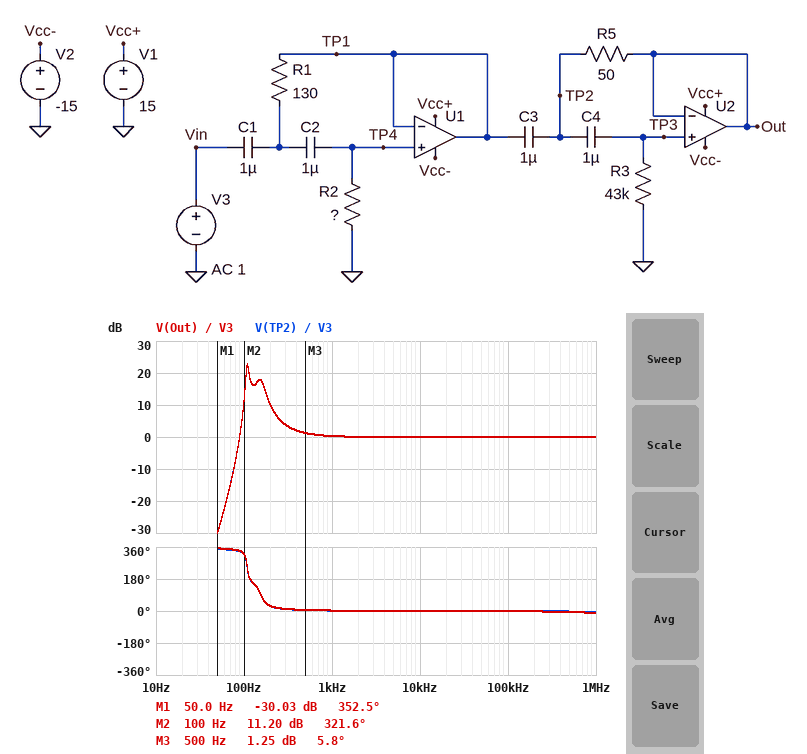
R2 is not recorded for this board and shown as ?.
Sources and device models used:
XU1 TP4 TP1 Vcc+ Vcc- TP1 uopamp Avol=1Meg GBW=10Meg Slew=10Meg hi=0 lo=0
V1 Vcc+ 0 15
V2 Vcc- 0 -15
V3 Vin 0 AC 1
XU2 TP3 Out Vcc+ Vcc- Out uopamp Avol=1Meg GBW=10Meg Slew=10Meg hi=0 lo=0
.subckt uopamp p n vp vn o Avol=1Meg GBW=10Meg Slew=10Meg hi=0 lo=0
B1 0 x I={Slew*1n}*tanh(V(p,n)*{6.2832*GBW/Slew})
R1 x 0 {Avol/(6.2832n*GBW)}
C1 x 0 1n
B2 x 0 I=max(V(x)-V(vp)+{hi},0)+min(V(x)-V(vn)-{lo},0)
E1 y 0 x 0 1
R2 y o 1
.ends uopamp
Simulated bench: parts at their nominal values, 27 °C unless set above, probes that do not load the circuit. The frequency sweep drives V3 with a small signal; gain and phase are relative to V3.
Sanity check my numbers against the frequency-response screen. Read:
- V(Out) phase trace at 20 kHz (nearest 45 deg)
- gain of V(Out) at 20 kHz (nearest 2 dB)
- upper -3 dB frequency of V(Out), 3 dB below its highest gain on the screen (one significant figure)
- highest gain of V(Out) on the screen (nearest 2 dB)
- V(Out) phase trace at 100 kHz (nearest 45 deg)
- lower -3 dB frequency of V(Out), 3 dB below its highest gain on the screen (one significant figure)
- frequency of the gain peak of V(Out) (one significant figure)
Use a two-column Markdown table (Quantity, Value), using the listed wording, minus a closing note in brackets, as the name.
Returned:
| Quantity | Value |
|---|---|
| V(Out) phase trace at 20 kHz | 0 deg |
| gain of V(Out) at 20 kHz | 0 dB |
| upper -3 dB frequency of V(Out), 3 dB below its highest gain on the screen | 100 Hz |
| highest gain of V(Out) on the screen | 22 dB |
| V(Out) phase trace at 100 kHz | 0 deg |
| lower -3 dB frequency of V(Out), 3 dB below its highest gain on the screen | 100 Hz |
| frequency of the gain peak of V(Out) | 100 Hz |
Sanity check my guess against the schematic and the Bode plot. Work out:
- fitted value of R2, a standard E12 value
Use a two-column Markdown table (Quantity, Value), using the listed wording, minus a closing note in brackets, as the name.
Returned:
| Quantity | Value |
|---|---|
| fitted value of R2, a standard E12 value | 8.2 kΩ |
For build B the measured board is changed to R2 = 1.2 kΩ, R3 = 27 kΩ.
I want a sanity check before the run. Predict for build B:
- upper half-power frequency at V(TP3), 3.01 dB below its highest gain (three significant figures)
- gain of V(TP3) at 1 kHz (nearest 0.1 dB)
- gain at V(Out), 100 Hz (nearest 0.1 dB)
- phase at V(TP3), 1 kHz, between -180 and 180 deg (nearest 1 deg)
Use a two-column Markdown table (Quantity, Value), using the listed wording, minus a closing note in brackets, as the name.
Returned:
| Quantity | Value |
|---|---|
| upper half-power frequency at V(TP3), 3.01 dB below its highest gain | 810 Hz |
| gain of V(TP3) at 1 kHz | 1.3 dB |
| gain at V(Out), 100 Hz | -22.7 dB |
| phase at V(TP3), 1 kHz, between -180 and 180 deg | 18 deg |
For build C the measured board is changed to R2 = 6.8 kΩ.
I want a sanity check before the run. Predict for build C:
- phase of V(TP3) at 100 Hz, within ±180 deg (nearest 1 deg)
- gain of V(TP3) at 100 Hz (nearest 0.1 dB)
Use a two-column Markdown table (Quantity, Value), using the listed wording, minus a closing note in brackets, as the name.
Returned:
| Quantity | Value |
|---|---|
| phase of V(TP3) at 100 Hz, within ±180 deg | -37 deg |
| gain of V(TP3) at 100 Hz | 8.6 dB |
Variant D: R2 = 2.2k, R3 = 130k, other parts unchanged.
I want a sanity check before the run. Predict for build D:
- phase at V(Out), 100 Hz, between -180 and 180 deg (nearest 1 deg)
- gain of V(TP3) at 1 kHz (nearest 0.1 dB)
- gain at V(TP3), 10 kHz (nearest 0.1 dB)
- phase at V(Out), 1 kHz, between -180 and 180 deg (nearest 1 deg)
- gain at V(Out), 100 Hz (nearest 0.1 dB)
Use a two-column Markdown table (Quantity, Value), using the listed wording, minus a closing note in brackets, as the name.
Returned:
| Quantity | Value |
|---|---|
| phase at V(Out), 100 Hz, between -180 and 180 deg | 172 deg |
| gain of V(TP3) at 1 kHz | 0.7 dB |
| gain at V(TP3), 10 kHz | 0 dB |
| phase at V(Out), 1 kHz, between -180 and 180 deg | 9 deg |
| gain at V(Out), 100 Hz | -13.8 dB |
